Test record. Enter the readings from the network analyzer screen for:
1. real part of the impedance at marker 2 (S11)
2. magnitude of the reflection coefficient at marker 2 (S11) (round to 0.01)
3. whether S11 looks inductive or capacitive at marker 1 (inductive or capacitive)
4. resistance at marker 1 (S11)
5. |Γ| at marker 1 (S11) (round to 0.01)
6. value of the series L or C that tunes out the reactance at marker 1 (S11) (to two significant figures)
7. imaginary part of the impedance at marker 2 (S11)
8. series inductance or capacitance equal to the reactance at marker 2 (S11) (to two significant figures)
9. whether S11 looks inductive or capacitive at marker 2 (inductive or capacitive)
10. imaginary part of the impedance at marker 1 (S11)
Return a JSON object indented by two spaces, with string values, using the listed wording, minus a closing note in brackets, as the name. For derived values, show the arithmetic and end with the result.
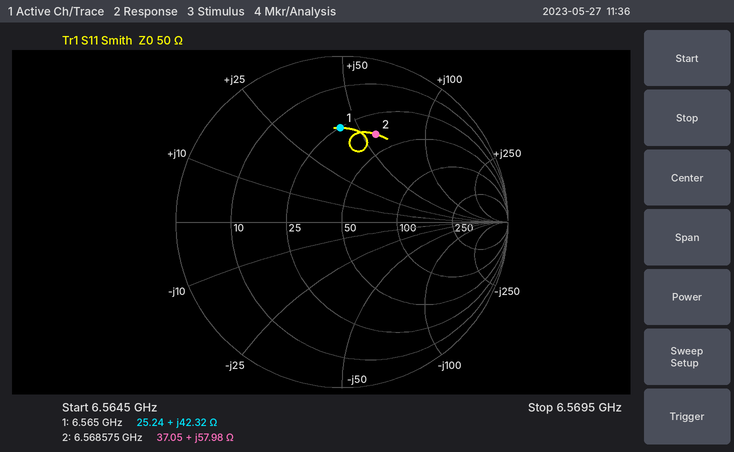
{
  "real part of the impedance at marker 2": "37.05 Ω",
  "magnitude of the reflection coefficient at marker 2 (S11)": "0.57",
  "whether S11 looks inductive or capacitive at marker 1": "inductive",
  "resistance at marker 1": "25.24 Ω",
  "|Γ| at marker 1 (S11)": "0.57",
  "value of the series L or C that tunes out the reactance at marker 1 (S11)": "C = 1/(2π × 6.565 GHz × 42.32 Ω) ≈ 573 fF, so 570 fF to two significant figures",
  "imaginary part of the impedance at marker 2": "+57.98 Ω",
  "series inductance or capacitance equal to the reactance at marker 2 (S11)": "L = 57.98 Ω/(2π × 6.568575 GHz) ≈ 1.4 nH",
  "whether S11 looks inductive or capacitive at marker 2": "inductive",
  "imaginary part of the impedance at marker 1": "+42.32 Ω"
}
